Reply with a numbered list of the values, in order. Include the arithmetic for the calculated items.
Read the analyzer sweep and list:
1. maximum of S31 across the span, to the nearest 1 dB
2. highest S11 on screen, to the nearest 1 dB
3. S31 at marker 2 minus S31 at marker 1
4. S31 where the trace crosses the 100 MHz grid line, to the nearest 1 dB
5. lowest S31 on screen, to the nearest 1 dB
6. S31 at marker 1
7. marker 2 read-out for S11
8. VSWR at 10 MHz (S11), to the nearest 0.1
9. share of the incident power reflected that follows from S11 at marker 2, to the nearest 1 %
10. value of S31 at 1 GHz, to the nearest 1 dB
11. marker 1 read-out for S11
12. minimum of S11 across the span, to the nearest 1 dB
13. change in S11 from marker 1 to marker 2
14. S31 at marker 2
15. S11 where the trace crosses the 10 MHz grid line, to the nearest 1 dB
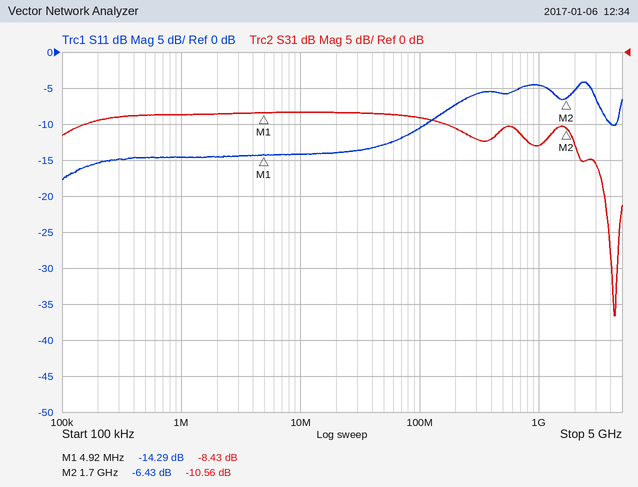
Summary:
1. -8 dB
2. -4 dB
3. -10.56 − (-8.43) = -2.13 dB
4. -9 dB
5. -37 dB
6. -8.43 dB
7. -6.43 dB
8. |Γ| = 10^(-14/20) = 0.1995; VSWR = (1 + 0.1995)/(1 − 0.1995) ≈ 1.5
9. 10^(-6.43/10) ≈ 23 %
10. -13 dB
11. -14.29 dB
12. -18 dB
13. -6.43 − (-14.29) = 7.86 dB
14. -10.56 dB
15. -14 dB
